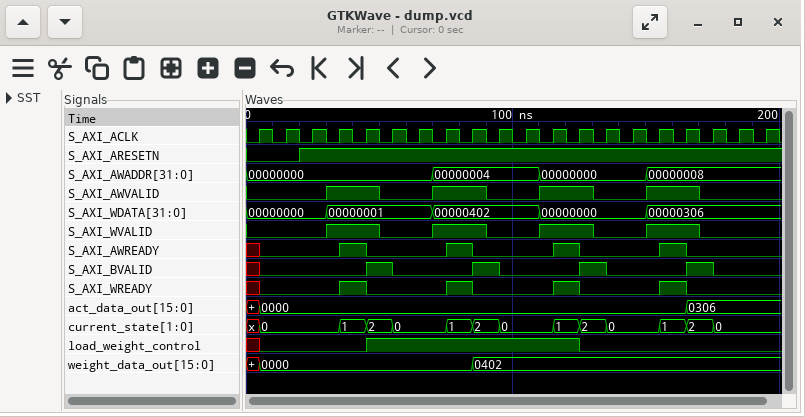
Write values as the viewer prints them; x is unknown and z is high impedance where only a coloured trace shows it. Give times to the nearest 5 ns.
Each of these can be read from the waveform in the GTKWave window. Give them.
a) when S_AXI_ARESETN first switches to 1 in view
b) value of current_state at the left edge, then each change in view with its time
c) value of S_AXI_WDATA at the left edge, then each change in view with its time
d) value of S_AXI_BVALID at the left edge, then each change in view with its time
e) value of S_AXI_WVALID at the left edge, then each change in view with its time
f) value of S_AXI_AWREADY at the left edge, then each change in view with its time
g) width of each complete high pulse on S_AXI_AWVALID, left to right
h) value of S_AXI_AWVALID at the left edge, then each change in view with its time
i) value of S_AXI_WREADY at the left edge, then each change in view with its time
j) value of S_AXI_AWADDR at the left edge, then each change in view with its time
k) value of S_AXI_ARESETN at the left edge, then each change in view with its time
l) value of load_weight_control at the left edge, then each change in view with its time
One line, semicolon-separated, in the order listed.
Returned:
20 ns; x, 0 at 5 ns, 1 at 35 ns, 2 at 45 ns, 0 at 55 ns, 1 at 75 ns, 2 at 85 ns, 0 at 95 ns, 1 at 115 ns, 2 at 125 ns, 0 at 135 ns, 1 at 155 ns, 2 at 165 ns, 0 at 175 ns; 00000000, 00000001 at 30 ns, 00000402 at 70 ns, 00000000 at 110 ns, 00000306 at 150 ns; x, 0 at 5 ns, 1 at 45 ns, 0 at 55 ns, 1 at 85 ns, 0 at 95 ns, 1 at 125 ns, 0 at 135 ns, 1 at 165 ns, 0 at 175 ns; 0, 1 at 30 ns, 0 at 50 ns, 1 at 70 ns, 0 at 90 ns, 1 at 110 ns, 0 at 130 ns, 1 at 150 ns, 0 at 170 ns; x, 0 at 5 ns, 1 at 35 ns, 0 at 45 ns, 1 at 75 ns, 0 at 85 ns, 1 at 115 ns, 0 at 125 ns, 1 at 155 ns, 0 at 165 ns; 20 ns, 20 ns, 20 ns, 20 ns; 0, 1 at 30 ns, 0 at 50 ns, 1 at 70 ns, 0 at 90 ns, 1 at 110 ns, 0 at 130 ns, 1 at 150 ns, 0 at 170 ns; x, 0 at 5 ns, 1 at 35 ns, 0 at 45 ns, 1 at 75 ns, 0 at 85 ns, 1 at 115 ns, 0 at 125 ns, 1 at 155 ns, 0 at 165 ns; 00000000, 00000004 at 70 ns, 00000000 at 110 ns, 00000008 at 150 ns; 0, 1 at 20 ns; x, 0 at 5 ns, 1 at 45 ns, 0 at 125 ns
